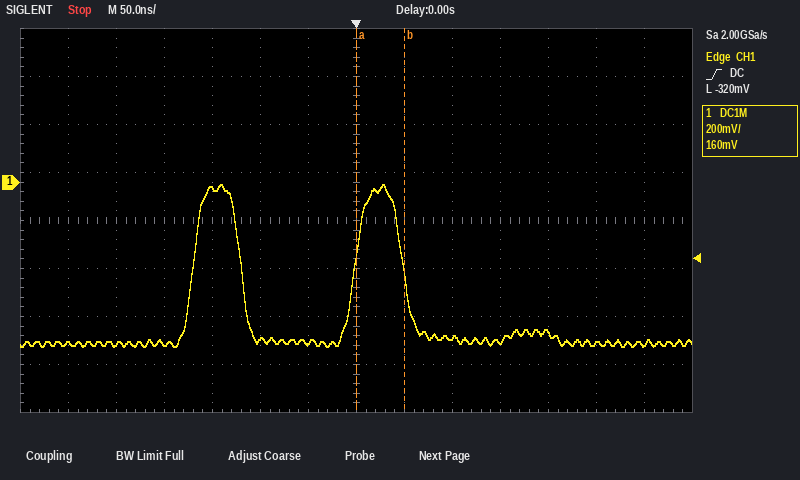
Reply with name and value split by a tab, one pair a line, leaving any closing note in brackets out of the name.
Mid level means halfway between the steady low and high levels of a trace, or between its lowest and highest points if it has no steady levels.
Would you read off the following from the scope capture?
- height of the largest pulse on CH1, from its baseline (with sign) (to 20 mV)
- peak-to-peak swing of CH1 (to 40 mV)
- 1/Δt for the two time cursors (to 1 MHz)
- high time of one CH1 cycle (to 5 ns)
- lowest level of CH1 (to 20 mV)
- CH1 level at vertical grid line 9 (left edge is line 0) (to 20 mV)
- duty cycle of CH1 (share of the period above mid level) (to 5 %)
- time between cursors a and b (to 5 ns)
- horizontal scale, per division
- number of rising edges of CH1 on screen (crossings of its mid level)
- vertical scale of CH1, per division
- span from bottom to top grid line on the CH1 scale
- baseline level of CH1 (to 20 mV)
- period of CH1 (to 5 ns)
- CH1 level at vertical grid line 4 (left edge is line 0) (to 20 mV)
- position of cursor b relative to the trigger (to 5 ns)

height of the largest pulse on CH1, from its baseline (with sign)	+660 mV
peak-to-peak swing of CH1	680 mV
1/Δt for the two time cursors	20 MHz
high time of one CH1 cycle	50 ns
lowest level of CH1	-680 mV
CH1 level at vertical grid line 9 (left edge is line 0)	-640 mV
duty cycle of CH1 (share of the period above mid level)	30 %
time between cursors a and b	50 ns
horizontal scale, per division	50 ns
number of rising edges of CH1 on screen	2
vertical scale of CH1, per division	200 mV
span from bottom to top grid line on the CH1 scale	1.6 V
baseline level of CH1	-660 mV
period of CH1	170 ns
CH1 level at vertical grid line 4 (left edge is line 0)	-20 mV
position of cursor b relative to the trigger	+50 ns
